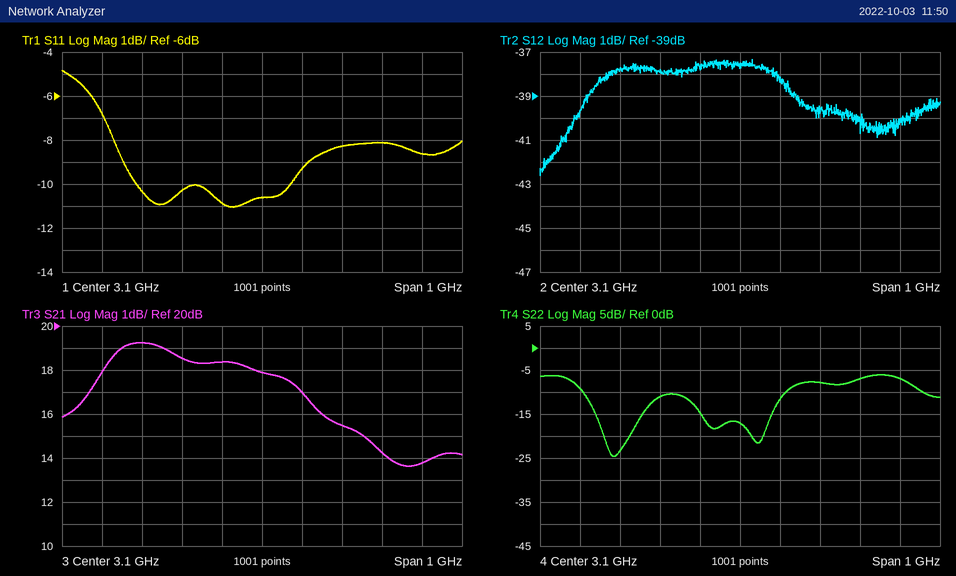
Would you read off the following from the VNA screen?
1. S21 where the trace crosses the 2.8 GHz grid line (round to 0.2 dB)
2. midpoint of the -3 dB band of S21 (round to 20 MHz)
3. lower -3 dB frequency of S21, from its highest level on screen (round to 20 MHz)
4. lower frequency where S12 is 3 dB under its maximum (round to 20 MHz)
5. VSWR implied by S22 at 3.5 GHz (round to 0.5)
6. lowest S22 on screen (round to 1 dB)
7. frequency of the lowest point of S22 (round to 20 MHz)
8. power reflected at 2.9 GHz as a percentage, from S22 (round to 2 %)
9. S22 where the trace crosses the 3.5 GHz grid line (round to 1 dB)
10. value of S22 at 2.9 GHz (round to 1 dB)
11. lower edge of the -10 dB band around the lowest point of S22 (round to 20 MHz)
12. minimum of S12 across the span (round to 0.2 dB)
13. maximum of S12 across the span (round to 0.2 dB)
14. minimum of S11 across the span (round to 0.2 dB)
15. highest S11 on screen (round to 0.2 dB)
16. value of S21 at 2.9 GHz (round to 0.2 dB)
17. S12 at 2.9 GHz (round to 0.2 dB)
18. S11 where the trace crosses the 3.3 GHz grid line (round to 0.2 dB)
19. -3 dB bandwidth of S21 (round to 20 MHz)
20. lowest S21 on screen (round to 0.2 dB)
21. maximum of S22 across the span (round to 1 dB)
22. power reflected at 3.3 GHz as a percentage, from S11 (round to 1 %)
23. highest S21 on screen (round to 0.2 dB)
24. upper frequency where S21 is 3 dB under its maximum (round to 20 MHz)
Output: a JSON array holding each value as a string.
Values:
["19.2 dB", "2.94 GHz", "2.64 GHz", "2.68 GHz", "2.5", "-25 dB", "2.78 GHz", "8 %", "-7 dB", "-11 dB", "2.70 GHz", "-42.6 dB", "-37.4 dB", "-11.0 dB", "-4.8 dB", "18.6 dB", "-37.8 dB", "-8.2 dB", "600 MHz", "13.6 dB", "-6 dB", "15 %", "19.2 dB", "3.24 GHz"]
